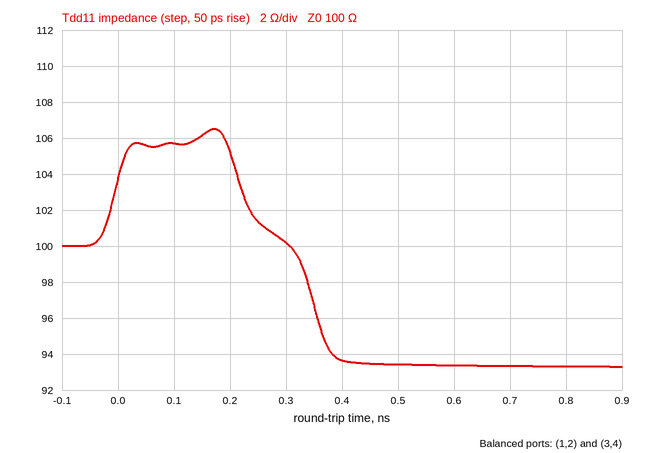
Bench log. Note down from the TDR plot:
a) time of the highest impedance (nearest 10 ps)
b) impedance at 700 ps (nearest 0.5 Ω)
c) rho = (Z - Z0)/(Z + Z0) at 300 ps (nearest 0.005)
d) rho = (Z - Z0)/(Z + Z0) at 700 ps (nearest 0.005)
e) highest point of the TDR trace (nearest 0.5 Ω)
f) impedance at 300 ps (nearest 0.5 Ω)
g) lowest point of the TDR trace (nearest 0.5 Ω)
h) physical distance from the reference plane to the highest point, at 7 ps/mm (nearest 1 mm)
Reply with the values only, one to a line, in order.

170 ps
93.5 Ω
0.000
-0.035
106.5 Ω
100.0 Ω
93.5 Ω
12 mm
